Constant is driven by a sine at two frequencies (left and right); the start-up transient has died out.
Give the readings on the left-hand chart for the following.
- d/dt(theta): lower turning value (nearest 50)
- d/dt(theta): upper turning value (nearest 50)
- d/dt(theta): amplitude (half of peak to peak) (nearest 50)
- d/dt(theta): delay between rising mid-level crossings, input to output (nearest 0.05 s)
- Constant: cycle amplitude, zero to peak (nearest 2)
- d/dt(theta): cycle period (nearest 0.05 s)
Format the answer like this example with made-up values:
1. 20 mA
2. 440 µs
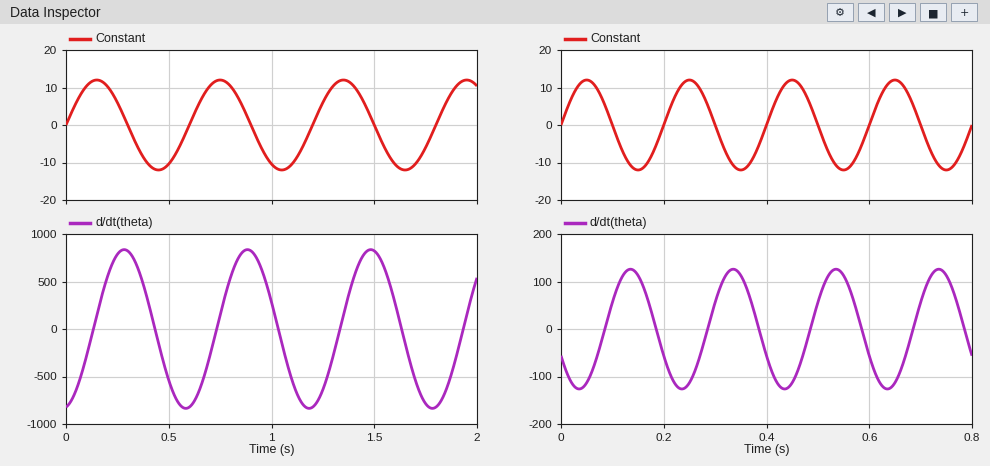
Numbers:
1. -850
2. 850
3. 850
4. 0.15 s
5. 12
6. 0.60 s
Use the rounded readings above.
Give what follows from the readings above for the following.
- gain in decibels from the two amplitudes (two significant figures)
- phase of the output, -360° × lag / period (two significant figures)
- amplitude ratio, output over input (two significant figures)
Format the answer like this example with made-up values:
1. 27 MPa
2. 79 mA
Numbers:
1. 37 dB
2. -90°
3. 71
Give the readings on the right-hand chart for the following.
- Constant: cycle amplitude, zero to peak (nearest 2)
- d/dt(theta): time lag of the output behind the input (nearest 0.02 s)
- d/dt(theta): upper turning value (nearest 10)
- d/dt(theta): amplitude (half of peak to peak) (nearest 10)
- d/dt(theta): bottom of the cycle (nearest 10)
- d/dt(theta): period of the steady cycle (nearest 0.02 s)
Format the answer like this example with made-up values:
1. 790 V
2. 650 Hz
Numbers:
1. 12
2. 0.08 s
3. 130
4. 130
5. -130
6. 0.20 s
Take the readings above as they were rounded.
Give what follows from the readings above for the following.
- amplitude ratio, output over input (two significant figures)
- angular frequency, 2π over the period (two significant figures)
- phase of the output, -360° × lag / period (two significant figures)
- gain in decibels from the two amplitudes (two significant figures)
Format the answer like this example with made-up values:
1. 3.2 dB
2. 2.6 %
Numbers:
1. 11
2. 31 rad/s
3. -140°
4. 21 dB
